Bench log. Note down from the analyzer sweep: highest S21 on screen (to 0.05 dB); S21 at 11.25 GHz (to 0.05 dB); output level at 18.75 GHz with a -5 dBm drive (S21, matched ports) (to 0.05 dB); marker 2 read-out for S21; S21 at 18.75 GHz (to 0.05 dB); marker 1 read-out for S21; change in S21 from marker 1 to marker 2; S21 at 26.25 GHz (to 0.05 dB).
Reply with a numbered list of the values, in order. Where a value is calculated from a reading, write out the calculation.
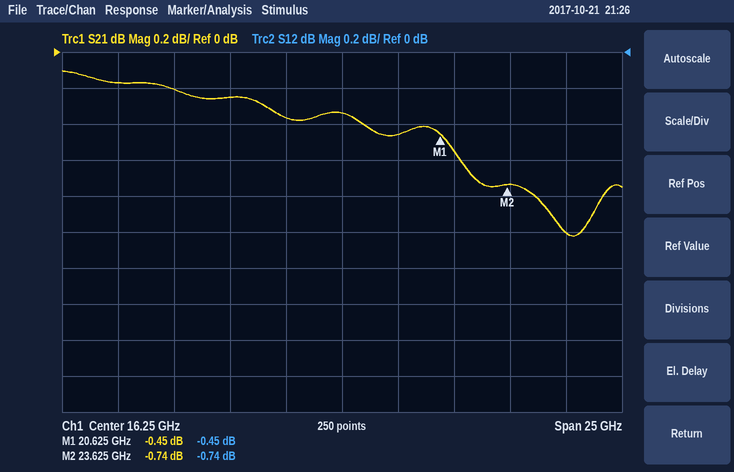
1. -0.10 dB
2. -0.25 dB
3. -5 dBm + (-0.45 dB) = -5.45 dBm
4. -0.74 dB
5. -0.45 dB
6. -0.45 dB
7. -0.74 − (-0.45) = -0.29 dB
8. -1.00 dB
